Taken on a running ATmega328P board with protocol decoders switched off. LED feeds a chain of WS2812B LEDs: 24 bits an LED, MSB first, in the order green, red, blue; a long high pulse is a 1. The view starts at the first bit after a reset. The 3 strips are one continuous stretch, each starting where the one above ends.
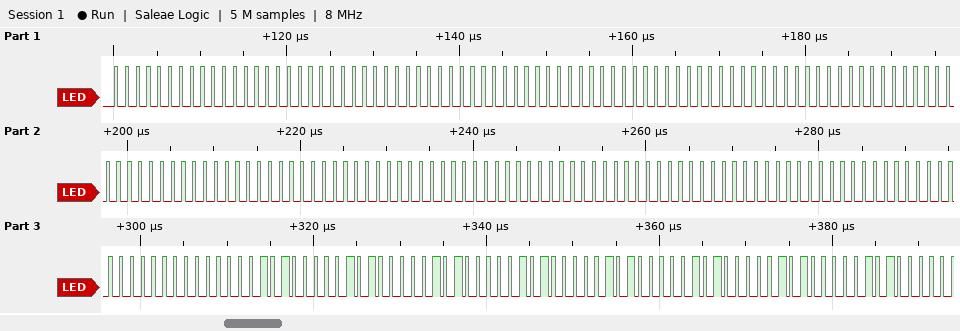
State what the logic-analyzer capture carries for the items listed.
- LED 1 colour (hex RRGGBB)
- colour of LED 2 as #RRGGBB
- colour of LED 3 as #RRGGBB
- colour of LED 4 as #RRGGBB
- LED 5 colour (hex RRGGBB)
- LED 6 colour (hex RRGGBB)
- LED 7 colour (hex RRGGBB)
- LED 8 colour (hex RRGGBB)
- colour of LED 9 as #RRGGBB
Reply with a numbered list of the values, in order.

1. #000000
2. #000000
3. #000000
4. #000000
5. #000000
6. #000000
7. #000000
8. #141414
9. #141414
